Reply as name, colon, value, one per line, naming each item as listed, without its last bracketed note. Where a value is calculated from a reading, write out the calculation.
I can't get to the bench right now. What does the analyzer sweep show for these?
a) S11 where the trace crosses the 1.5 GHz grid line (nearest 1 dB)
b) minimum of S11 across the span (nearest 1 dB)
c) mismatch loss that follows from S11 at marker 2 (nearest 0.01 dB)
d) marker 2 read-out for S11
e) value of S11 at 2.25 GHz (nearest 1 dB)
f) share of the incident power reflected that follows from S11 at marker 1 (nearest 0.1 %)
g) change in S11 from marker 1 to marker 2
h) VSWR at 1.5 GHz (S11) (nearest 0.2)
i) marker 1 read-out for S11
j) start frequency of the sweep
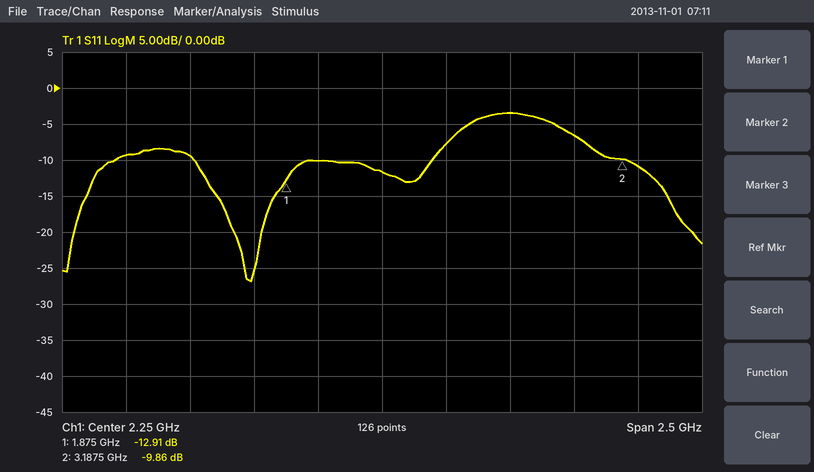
S11 where the trace crosses the 1.5 GHz grid line: -9 dB
minimum of S11 across the span: -27 dB
mismatch loss that follows from S11 at marker 2: −10 log10(1 − 10^(-9.86/10)) ≈ 0.47 dB
marker 2 read-out for S11: -9.86 dB
value of S11 at 2.25 GHz: -12 dB
share of the incident power reflected that follows from S11 at marker 1: 10^(-12.91/10) ≈ 5.1 %
change in S11 from marker 1 to marker 2: -9.86 − (-12.91) = 3.05 dB
VSWR at 1.5 GHz (S11): |Γ| = 10^(-9/20) = 0.3548; VSWR = (1 + 0.3548)/(1 − 0.3548) ≈ 2.10, so 2.0 to the nearest 0.2
marker 1 read-out for S11: -12.91 dB
start frequency of the sweep: 1 GHz
